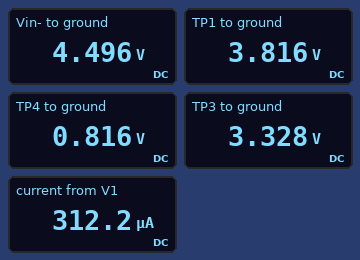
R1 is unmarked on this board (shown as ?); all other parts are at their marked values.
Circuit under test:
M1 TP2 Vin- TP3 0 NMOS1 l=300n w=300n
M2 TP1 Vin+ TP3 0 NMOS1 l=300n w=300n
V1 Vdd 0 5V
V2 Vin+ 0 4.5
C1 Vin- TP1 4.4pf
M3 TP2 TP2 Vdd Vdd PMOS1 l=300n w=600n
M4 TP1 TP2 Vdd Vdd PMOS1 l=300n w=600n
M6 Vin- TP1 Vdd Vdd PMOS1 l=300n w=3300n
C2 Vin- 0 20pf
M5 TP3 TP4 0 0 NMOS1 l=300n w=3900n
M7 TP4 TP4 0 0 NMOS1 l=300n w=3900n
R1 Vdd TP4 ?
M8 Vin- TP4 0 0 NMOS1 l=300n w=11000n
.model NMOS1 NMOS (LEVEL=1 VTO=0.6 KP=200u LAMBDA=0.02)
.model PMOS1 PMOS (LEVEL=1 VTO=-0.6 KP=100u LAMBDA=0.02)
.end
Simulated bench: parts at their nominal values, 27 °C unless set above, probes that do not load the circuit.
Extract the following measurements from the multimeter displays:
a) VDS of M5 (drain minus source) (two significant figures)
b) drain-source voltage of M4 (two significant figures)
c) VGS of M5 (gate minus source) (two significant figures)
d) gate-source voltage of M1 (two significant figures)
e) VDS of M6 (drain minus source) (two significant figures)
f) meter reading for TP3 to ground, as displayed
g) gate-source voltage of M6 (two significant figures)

3.3 V
-1.2 V
820 mV
1.2 V
-500 mV
3.328 V
-1.2 V
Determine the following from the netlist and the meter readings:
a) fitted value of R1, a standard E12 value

68 kΩ
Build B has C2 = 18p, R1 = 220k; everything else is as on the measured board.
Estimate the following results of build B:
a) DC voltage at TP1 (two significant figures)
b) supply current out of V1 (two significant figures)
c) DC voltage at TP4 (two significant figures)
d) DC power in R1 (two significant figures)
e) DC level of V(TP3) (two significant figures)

4.1 V
99 µA
720 mV
83 µW
3.6 V
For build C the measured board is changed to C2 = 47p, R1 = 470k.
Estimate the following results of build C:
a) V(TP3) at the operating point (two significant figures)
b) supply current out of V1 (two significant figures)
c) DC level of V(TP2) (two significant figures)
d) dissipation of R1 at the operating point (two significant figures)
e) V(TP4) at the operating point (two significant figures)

3.7 V
47 µA
4.2 V
40 µW
680 mV
